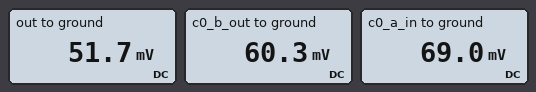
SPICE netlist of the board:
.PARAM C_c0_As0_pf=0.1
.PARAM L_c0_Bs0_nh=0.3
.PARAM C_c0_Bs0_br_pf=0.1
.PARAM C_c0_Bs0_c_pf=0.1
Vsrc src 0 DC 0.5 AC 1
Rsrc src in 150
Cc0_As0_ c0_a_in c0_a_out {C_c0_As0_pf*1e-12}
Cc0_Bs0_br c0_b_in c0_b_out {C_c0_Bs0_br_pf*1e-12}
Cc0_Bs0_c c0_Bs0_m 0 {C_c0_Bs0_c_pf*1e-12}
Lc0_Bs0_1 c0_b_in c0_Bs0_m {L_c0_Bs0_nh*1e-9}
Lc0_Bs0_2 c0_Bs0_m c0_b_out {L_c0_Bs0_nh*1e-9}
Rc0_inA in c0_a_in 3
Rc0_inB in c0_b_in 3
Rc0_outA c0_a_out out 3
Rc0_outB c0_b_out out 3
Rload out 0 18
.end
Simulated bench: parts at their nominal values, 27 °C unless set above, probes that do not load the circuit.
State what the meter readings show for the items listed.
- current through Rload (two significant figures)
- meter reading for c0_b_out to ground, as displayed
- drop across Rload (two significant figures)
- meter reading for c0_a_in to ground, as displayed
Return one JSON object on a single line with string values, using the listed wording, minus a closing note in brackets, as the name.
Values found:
{"current through Rload": "2.9 mA", "meter reading for c0_b_out to ground, as displayed": "60.3 mV", "drop across Rload": "52 mV", "meter reading for c0_a_in to ground, as displayed": "69.0 mV"}
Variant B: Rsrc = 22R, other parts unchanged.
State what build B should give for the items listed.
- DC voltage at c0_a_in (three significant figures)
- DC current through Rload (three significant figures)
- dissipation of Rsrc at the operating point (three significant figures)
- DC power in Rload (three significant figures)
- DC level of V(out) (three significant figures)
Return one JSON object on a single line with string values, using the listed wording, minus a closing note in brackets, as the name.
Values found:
{"DC voltage at c0_a_in": "261 mV", "DC current through Rload": "10.9 mA", "dissipation of Rsrc at the operating point": "2.60 mW", "DC power in Rload": "2.13 mW", "DC level of V(out)": "196 mV"}
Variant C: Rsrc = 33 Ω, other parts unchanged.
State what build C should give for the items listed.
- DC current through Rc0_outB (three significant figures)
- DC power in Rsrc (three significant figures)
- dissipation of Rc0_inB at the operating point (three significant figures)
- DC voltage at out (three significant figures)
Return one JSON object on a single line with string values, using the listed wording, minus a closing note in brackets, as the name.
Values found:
{"DC current through Rc0_outB": "8.77 mA", "DC power in Rsrc": "2.54 mW", "dissipation of Rc0_inB at the operating point": "231 µW", "DC voltage at out": "158 mV"}
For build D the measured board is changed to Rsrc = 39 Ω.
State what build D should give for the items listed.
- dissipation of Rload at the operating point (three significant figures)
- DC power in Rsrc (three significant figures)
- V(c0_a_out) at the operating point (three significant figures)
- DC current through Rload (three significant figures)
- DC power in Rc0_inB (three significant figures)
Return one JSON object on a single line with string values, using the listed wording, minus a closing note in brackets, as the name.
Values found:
{"dissipation of Rload at the operating point": "1.13 mW", "DC power in Rsrc": "2.46 mW", "V(c0_a_out) at the operating point": "143 mV", "DC current through Rload": "7.94 mA", "DC power in Rc0_inB": "189 µW"}
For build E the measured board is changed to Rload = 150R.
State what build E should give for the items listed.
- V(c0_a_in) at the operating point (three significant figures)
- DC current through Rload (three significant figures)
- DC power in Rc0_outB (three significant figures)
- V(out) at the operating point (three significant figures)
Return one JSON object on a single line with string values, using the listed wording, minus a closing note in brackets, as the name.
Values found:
{"V(c0_a_in) at the operating point": "255 mV", "DC current through Rload": "1.63 mA", "DC power in Rc0_outB": "8.01 µW", "V(out) at the operating point": "245 mV"}
